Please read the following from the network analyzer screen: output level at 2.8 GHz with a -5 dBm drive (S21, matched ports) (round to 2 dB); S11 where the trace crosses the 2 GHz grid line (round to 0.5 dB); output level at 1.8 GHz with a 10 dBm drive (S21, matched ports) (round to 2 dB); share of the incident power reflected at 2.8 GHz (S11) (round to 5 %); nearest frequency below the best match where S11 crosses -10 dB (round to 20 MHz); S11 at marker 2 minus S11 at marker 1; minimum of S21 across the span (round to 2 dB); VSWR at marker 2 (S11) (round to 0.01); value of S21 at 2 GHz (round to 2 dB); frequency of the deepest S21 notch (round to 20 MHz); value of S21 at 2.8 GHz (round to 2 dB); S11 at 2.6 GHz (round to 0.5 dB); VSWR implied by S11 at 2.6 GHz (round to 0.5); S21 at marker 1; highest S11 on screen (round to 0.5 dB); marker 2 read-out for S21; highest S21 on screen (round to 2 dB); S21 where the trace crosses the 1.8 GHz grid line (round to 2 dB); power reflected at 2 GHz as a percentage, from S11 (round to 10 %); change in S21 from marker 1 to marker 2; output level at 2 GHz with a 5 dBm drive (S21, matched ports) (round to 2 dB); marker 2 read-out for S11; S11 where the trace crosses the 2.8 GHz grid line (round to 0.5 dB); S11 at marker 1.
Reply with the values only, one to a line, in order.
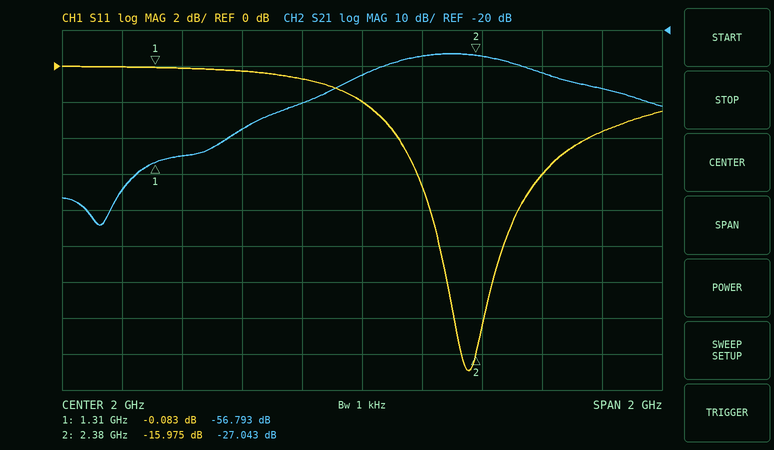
-42 dBm
-2.0 dB
-30 dBm
45 %
2.26 GHz
-15.892 dB
-74 dB
1.38
-32 dB
1.12 GHz
-36 dB
-6.0 dB
3.0
-56.793 dB
0.0 dB
-27.043 dB
-26 dB
-40 dB
60 %
29.750 dB
-28 dBm
-15.975 dB
-3.5 dB
-0.083 dB
